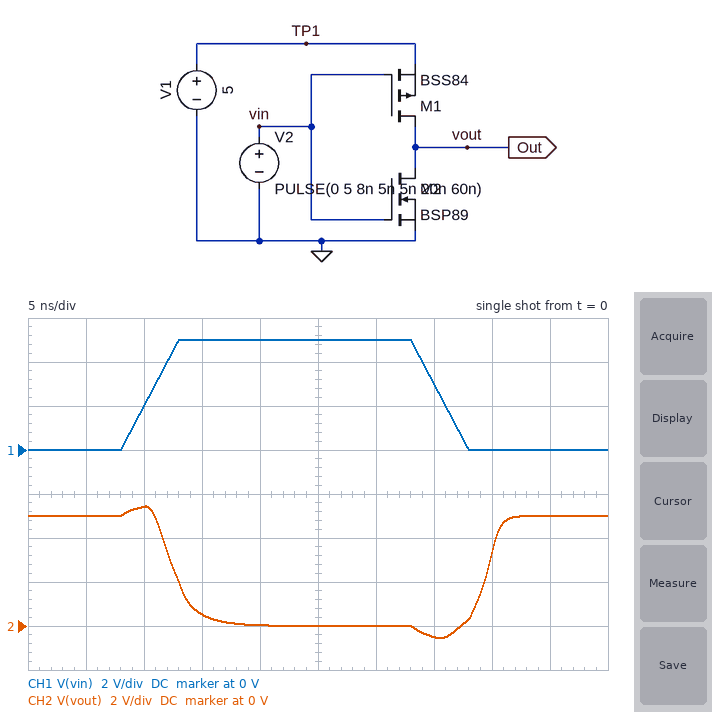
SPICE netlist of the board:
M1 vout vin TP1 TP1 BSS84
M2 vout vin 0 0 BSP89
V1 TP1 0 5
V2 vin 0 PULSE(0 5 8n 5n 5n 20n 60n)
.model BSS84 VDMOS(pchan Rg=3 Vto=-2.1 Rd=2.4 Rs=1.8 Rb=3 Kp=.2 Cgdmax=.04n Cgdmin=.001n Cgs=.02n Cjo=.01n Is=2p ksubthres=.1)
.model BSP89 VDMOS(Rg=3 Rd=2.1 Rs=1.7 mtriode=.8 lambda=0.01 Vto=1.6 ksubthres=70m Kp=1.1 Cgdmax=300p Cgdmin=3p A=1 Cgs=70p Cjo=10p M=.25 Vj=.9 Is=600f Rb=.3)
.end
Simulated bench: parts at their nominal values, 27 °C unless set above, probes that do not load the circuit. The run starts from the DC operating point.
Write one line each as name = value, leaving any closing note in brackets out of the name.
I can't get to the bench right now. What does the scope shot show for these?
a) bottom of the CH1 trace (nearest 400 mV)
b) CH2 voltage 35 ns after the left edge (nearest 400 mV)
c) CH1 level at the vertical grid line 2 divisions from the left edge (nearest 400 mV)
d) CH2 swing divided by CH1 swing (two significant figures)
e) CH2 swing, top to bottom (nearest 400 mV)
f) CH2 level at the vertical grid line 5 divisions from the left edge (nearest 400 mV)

bottom of the CH1 trace = 0 V
CH2 voltage 35 ns after the left edge = -400 mV
CH1 level at the vertical grid line 2 divisions from the left edge = 2.0 V
CH2 swing divided by CH1 swing = 1.2
CH2 swing, top to bottom = 6.0 V
CH2 level at the vertical grid line 5 divisions from the left edge = 0 V
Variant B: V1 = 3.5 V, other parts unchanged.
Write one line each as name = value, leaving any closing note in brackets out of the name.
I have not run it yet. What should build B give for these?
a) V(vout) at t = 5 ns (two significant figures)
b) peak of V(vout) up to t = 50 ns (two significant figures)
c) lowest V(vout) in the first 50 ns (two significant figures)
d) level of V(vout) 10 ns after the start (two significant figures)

V(vout) at t = 5 ns = 3.5 V
peak of V(vout) up to t = 50 ns = 4.3 V
lowest V(vout) in the first 50 ns = -670 mV
level of V(vout) 10 ns after the start = 4.2 V
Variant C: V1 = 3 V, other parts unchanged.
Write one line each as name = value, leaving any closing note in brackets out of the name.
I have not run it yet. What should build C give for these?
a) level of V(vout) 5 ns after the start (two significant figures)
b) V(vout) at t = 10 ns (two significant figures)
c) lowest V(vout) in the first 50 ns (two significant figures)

level of V(vout) 5 ns after the start = 3.0 V
V(vout) at t = 10 ns = 3.8 V
lowest V(vout) in the first 50 ns = -700 mV
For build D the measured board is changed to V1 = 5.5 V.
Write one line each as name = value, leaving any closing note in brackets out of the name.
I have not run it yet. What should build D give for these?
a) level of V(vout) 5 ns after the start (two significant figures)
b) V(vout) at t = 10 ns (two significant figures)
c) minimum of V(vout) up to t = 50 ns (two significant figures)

level of V(vout) 5 ns after the start = 5.5 V
V(vout) at t = 10 ns = 5.9 V
minimum of V(vout) up to t = 50 ns = -490 mV
